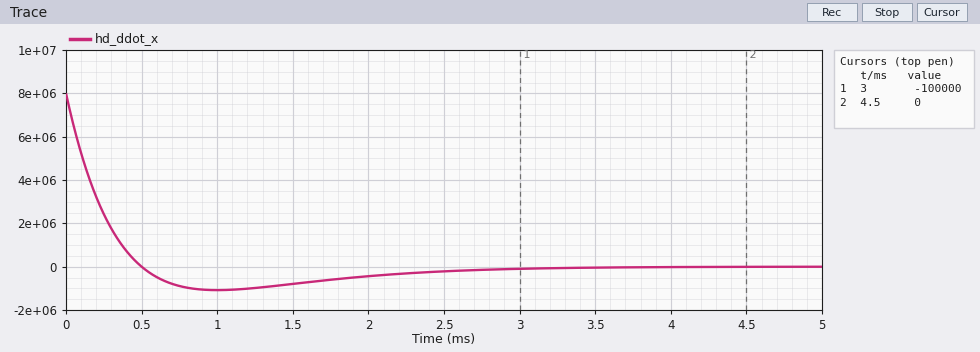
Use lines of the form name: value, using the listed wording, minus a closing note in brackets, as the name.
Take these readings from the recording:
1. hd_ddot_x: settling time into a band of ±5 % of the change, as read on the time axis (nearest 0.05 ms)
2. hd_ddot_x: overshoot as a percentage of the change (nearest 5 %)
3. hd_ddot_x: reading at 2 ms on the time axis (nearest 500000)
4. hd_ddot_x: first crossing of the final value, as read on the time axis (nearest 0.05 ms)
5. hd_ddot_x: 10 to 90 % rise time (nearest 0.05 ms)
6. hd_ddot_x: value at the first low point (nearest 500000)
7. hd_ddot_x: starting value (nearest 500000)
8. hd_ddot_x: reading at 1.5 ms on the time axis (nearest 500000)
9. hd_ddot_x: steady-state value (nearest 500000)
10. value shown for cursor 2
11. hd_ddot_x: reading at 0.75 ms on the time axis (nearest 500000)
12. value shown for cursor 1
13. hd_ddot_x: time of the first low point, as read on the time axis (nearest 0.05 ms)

hd_ddot_x: settling time into a band of ±5 % of the change, as read on the time axis: 2.05 ms
hd_ddot_x: overshoot as a percentage of the change: 15 %
hd_ddot_x: reading at 2 ms on the time axis: -500000
hd_ddot_x: first crossing of the final value, as read on the time axis: 0.50 ms
hd_ddot_x: 10 to 90 % rise time: 0.35 ms
hd_ddot_x: value at the first low point: -1000000
hd_ddot_x: starting value: 8000000
hd_ddot_x: reading at 1.5 ms on the time axis: -1000000
hd_ddot_x: steady-state value: 0
value shown for cursor 2: 0
hd_ddot_x: reading at 0.75 ms on the time axis: -1000000
value shown for cursor 1: -100000
hd_ddot_x: time of the first low point, as read on the time axis: 1.00 ms
